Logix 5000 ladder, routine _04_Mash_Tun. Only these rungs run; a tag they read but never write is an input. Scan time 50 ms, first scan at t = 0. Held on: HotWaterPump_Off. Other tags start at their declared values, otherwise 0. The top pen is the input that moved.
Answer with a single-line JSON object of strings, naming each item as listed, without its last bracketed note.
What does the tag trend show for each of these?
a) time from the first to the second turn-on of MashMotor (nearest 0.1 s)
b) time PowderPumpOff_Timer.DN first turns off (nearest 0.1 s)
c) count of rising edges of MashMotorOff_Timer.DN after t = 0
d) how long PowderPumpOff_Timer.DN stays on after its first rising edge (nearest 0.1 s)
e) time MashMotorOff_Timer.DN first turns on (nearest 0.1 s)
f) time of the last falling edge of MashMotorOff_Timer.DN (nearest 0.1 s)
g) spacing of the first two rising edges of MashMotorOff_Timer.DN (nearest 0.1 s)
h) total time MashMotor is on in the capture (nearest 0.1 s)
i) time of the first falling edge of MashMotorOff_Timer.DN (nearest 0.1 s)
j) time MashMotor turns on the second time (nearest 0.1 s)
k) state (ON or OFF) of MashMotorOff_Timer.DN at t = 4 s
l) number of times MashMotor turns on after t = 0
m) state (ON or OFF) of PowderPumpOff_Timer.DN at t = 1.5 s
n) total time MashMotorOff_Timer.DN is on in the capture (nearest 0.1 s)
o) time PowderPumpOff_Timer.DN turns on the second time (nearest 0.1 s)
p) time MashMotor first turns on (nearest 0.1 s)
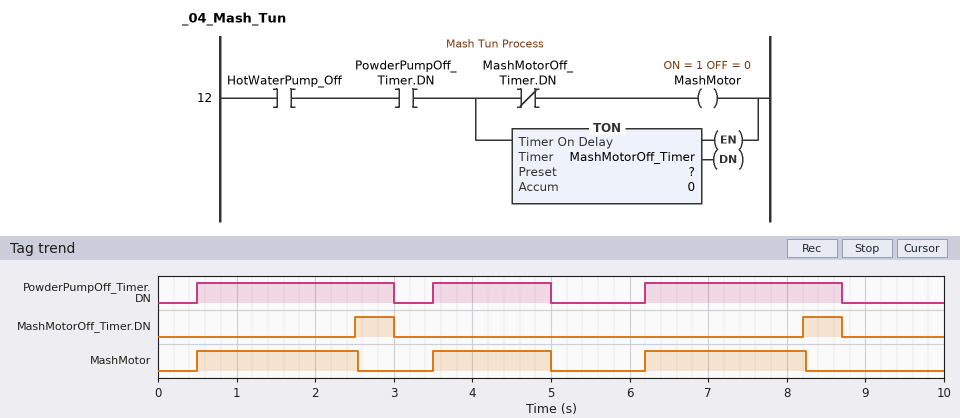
{"time from the first to the second turn-on of MashMotor": "3.0 s", "time PowderPumpOff_Timer.DN first turns off": "3.0 s", "count of rising edges of MashMotorOff_Timer.DN after t = 0": "2", "how long PowderPumpOff_Timer.DN stays on after its first rising edge": "2.5 s", "time MashMotorOff_Timer.DN first turns on": "2.5 s", "time of the last falling edge of MashMotorOff_Timer.DN": "8.7 s", "spacing of the first two rising edges of MashMotorOff_Timer.DN": "5.7 s", "total time MashMotor is on in the capture": "5.6 s", "time of the first falling edge of MashMotorOff_Timer.DN": "3.0 s", "time MashMotor turns on the second time": "3.5 s", "state (ON or OFF) of MashMotorOff_Timer.DN at t = 4 s": "OFF", "number of times MashMotor turns on after t = 0": "3", "state (ON or OFF) of PowderPumpOff_Timer.DN at t = 1.5 s": "ON", "total time MashMotorOff_Timer.DN is on in the capture": "1.0 s", "time PowderPumpOff_Timer.DN turns on the second time": "3.5 s", "time MashMotor first turns on": "0.5 s"}
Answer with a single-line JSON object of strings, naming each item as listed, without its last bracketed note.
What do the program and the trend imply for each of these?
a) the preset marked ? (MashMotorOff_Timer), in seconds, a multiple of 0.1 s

{"the preset marked ? (MashMotorOff_Timer), in seconds, a multiple of 0.1 s": "2.0 s"}
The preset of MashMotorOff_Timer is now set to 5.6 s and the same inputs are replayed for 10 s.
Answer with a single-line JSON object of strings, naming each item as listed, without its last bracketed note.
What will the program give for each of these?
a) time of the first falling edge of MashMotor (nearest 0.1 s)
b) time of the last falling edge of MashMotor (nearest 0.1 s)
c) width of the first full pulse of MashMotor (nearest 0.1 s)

{"time of the first falling edge of MashMotor": "3.0 s", "time of the last falling edge of MashMotor": "8.7 s", "width of the first full pulse of MashMotor": "2.5 s"}
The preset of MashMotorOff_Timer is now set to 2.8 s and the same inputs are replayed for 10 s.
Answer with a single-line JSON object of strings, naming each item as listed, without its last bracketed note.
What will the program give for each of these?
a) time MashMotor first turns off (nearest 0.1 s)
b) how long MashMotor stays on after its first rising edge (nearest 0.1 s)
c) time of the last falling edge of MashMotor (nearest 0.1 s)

{"time MashMotor first turns off": "3.0 s", "how long MashMotor stays on after its first rising edge": "2.5 s", "time of the last falling edge of MashMotor": "8.7 s"}
